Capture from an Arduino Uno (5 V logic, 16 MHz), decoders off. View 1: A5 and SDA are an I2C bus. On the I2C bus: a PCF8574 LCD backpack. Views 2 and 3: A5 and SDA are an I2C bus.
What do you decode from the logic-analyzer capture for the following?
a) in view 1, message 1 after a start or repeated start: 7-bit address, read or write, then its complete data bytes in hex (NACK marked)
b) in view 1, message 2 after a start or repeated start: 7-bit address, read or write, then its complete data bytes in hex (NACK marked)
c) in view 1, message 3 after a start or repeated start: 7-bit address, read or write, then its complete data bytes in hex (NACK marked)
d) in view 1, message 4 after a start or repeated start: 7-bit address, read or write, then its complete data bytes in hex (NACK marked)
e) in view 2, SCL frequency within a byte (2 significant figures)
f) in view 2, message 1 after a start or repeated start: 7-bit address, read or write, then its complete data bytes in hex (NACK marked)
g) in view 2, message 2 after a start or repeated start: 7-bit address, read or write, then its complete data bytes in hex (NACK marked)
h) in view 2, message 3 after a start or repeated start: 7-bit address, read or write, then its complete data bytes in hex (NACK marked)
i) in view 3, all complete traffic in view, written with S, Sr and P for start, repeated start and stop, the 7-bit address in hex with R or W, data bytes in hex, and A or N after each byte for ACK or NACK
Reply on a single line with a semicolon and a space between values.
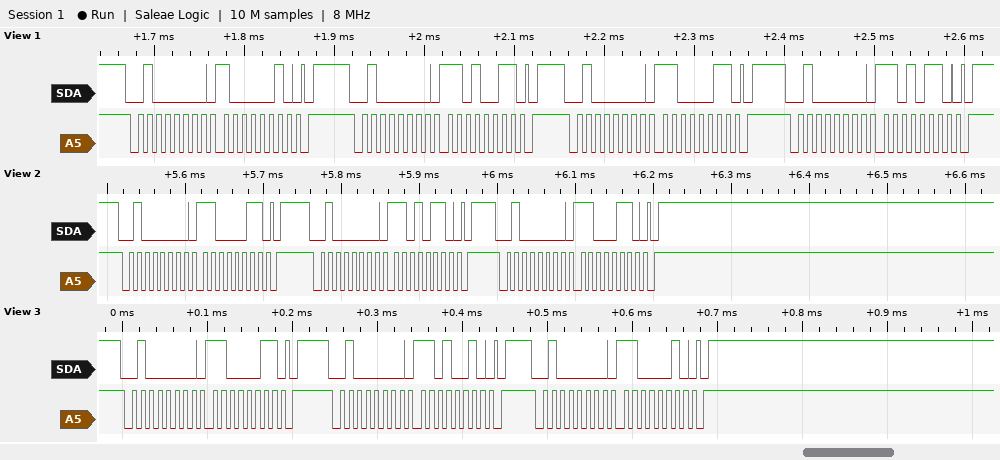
0x20 write: 82; 0x20 write: D3; 0x20 write: C3; 0x20 write: D6; 100 kHz; 0x20 write: C3; 0x20 write: D6; 0x20 write: C6; S 20W A C3 A P S 20W A D2 A P S 20W A C2 A P
